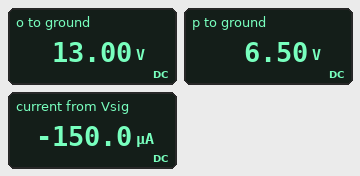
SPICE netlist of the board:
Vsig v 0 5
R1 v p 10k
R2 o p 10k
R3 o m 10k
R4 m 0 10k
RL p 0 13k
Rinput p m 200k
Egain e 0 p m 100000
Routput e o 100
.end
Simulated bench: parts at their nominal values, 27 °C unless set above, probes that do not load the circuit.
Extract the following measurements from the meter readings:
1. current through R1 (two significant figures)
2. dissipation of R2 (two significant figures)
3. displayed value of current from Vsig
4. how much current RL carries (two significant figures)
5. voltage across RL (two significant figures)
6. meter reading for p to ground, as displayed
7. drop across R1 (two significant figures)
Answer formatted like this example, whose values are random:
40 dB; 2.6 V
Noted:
150 µA; 4.2 mW; -150.0 µA; 500 µA; 6.5 V; 6.50 V; 1.5 V
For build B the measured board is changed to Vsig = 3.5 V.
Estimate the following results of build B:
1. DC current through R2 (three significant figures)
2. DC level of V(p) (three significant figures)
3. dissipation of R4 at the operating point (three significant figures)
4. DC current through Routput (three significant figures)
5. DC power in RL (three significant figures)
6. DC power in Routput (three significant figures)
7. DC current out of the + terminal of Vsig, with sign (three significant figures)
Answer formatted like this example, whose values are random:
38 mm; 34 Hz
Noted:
455 µA; 4.55 V; 2.07 mW; 910 µA; 1.59 mW; 82.8 µW; -105 µA
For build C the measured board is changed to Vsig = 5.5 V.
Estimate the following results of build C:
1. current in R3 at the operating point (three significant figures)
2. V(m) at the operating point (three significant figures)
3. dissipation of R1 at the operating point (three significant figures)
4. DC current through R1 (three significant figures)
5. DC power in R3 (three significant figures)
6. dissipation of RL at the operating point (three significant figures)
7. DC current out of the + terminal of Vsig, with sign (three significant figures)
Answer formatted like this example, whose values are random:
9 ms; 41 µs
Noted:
715 µA; 7.15 V; 272 µW; 165 µA; 5.11 mW; 3.93 mW; -165 µA
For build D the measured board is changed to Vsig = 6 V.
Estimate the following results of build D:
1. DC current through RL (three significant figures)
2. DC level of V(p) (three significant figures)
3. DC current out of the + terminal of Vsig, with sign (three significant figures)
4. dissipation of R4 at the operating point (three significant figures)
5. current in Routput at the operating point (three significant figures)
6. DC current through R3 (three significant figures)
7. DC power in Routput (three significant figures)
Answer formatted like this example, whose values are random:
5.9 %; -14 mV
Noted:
600 µA; 7.80 V; -180 µA; 6.08 mW; 1.56 mA; 780 µA; 243 µW
